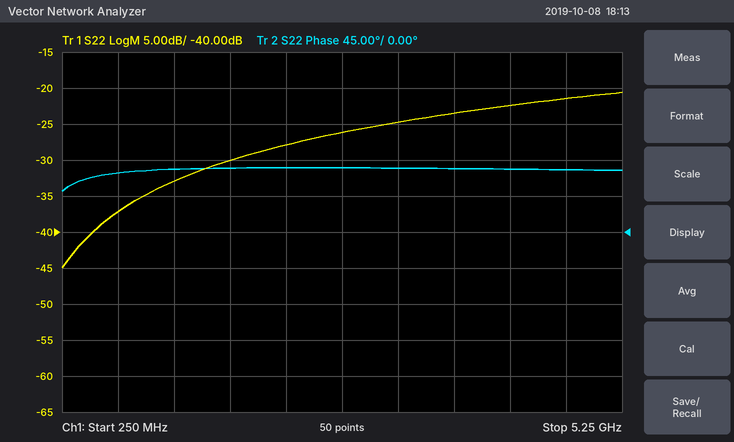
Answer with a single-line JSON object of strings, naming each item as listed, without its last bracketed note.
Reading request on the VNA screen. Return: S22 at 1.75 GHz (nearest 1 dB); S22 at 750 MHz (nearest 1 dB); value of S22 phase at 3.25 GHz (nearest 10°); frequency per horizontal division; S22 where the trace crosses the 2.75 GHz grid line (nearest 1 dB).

{"S22 at 1.75 GHz": "-30 dB", "S22 at 750 MHz": "-37 dB", "value of S22 phase at 3.25 GHz": "80°", "frequency per horizontal division": "500 MHz", "S22 where the trace crosses the 2.75 GHz grid line": "-26 dB"}
